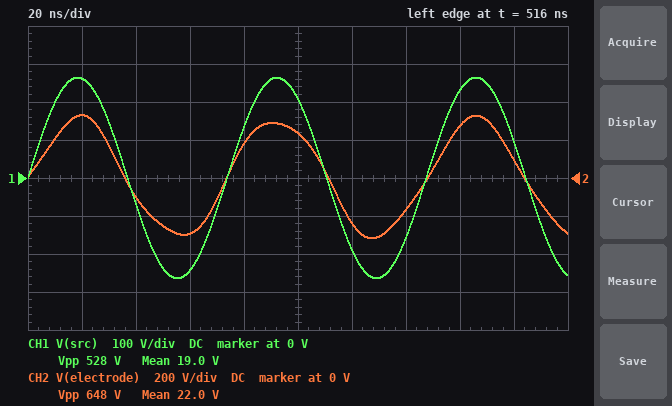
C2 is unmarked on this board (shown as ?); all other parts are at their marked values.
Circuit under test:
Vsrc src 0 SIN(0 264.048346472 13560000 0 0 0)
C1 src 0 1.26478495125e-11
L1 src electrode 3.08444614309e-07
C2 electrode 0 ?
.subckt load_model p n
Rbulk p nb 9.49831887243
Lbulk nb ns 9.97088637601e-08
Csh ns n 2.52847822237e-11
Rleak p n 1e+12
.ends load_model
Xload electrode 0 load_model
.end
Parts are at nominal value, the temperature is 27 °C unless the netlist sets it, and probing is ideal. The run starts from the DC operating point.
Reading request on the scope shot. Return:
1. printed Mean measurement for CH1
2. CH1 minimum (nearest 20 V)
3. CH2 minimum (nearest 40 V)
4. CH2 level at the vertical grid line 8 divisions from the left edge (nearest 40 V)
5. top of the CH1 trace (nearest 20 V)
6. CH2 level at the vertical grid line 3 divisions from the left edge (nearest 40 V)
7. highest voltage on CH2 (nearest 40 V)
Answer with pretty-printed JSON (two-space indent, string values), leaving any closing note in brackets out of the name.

{
  "printed Mean measurement for CH1": "19.0 V",
  "CH1 minimum": "-260 V",
  "CH2 minimum": "-320 V",
  "CH2 level at the vertical grid line 8 divisions from the left edge": "280 V",
  "top of the CH1 trace": "260 V",
  "CH2 level at the vertical grid line 3 divisions from the left edge": "-280 V",
  "highest voltage on CH2": "320 V"
}
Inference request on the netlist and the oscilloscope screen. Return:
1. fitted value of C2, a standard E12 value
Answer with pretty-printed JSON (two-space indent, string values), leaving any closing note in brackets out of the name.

{
  "fitted value of C2, a standard E12 value": "39 pF"
}
